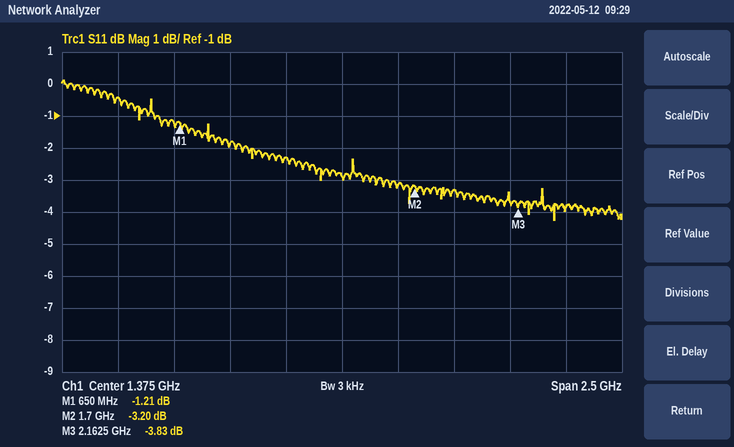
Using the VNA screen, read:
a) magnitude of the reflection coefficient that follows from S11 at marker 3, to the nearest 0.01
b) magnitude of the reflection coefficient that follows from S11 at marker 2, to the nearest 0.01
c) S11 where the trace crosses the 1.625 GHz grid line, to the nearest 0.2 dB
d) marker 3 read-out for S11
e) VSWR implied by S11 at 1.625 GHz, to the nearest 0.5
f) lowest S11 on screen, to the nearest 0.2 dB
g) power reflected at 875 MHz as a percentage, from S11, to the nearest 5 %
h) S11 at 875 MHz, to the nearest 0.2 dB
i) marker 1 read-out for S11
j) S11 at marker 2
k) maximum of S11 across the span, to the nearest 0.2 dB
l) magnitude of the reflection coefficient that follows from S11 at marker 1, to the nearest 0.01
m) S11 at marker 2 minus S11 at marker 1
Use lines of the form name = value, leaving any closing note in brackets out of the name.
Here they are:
magnitude of the reflection coefficient that follows from S11 at marker 3, to the nearest 0.01 = 0.64
magnitude of the reflection coefficient that follows from S11 at marker 2, to the nearest 0.01 = 0.69
S11 where the trace crosses the 1.625 GHz grid line, to the nearest 0.2 dB = -3.2 dB
marker 3 read-out for S11 = -3.83 dB
VSWR implied by S11 at 1.625 GHz, to the nearest 0.5 = 5.5
lowest S11 on screen, to the nearest 0.2 dB = -4.2 dB
power reflected at 875 MHz as a percentage, from S11, to the nearest 5 % = 65 %
S11 at 875 MHz, to the nearest 0.2 dB = -1.8 dB
marker 1 read-out for S11 = -1.21 dB
S11 at marker 2 = -3.20 dB
maximum of S11 across the span, to the nearest 0.2 dB = 0.2 dB
magnitude of the reflection coefficient that follows from S11 at marker 1, to the nearest 0.01 = 0.87
S11 at marker 2 minus S11 at marker 1 = -1.99 dB
